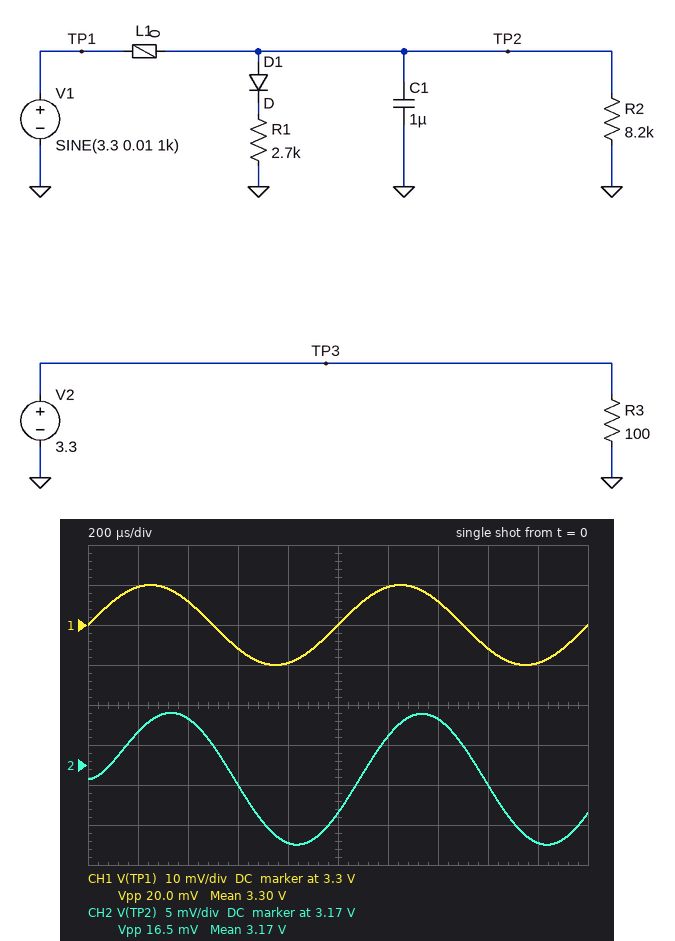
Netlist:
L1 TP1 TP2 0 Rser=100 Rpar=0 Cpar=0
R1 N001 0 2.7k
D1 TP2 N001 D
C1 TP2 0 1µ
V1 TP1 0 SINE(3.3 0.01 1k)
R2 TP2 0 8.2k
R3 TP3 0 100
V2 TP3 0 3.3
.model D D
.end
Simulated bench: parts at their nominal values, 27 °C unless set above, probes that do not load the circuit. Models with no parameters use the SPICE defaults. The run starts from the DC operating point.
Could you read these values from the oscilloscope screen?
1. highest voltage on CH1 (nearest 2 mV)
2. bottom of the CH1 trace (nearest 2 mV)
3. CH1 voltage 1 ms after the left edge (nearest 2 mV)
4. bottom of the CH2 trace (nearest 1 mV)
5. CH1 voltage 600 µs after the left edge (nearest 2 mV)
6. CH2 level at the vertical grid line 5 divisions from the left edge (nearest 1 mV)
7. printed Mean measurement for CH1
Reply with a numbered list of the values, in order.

1. 3.310 V
2. 3.290 V
3. 3.300 V
4. 3.160 V
5. 3.294 V
6. 3.164 V
7. 3.30 V
